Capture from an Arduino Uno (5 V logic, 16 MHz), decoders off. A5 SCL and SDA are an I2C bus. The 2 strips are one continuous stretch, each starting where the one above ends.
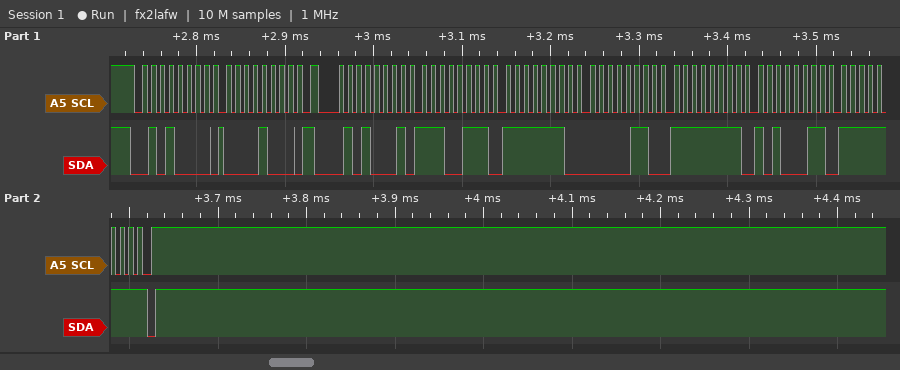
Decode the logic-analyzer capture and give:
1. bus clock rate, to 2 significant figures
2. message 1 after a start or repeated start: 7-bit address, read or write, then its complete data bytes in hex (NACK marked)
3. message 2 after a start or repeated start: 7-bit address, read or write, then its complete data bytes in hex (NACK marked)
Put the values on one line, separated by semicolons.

100 kHz; 0x28 write: 08; 0x28 read: E7 FE 06 FF A3 FF NACK
